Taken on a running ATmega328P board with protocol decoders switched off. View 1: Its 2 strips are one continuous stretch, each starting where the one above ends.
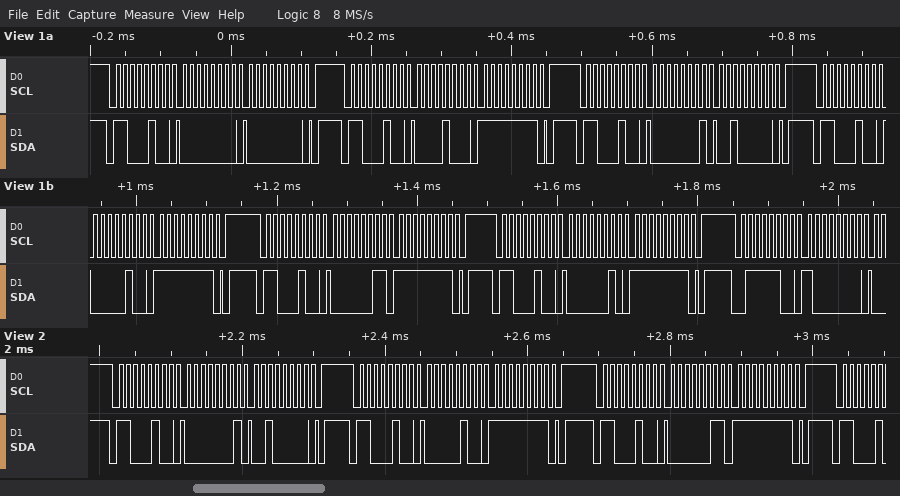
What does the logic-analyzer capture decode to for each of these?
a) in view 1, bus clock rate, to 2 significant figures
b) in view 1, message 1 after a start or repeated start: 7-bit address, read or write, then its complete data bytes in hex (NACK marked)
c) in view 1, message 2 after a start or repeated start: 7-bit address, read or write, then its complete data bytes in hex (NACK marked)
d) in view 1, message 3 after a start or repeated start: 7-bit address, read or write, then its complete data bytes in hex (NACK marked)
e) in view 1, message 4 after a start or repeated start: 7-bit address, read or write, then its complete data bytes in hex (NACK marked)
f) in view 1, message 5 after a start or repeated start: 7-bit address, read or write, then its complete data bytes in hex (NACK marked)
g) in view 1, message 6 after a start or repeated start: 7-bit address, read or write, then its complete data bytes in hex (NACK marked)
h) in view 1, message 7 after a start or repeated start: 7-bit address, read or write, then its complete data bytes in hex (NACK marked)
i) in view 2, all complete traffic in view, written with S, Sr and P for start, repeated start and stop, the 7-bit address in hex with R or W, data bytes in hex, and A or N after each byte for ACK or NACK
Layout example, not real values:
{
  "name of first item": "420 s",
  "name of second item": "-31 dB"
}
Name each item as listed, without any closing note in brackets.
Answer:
{
  "in view 1, bus clock rate, to 2 significant figures": "100 kHz",
  "in view 1, message 1 after a start or repeated start: 7-bit address, read or write, then its complete data bytes in hex": "0x62 write: 00 00",
  "in view 1, message 2 after a start or repeated start: 7-bit address, read or write, then its complete data bytes in hex": "0x62 write: 08 FF",
  "in view 1, message 3 after a start or repeated start: 7-bit address, read or write, then its complete data bytes in hex": "0x62 write: 01 20",
  "in view 1, message 4 after a start or repeated start: 7-bit address, read or write, then its complete data bytes in hex": "0x62 write: 04 FF",
  "in view 1, message 5 after a start or repeated start: 7-bit address, read or write, then its complete data bytes in hex": "0x62 write: 03 FF",
  "in view 1, message 6 after a start or repeated start: 7-bit address, read or write, then its complete data bytes in hex": "0x62 write: 02 FF",
  "in view 1, message 7 after a start or repeated start: 7-bit address, read or write, then its complete data bytes in hex": "0x3E write: 80",
  "in view 2, all complete traffic in view, written with S, Sr and P for start, repeated start and stop, the 7-bit address in hex with R or W, data bytes in hex, and A or N after each byte for ACK or NACK": "S 62W A 01 A 20 A P S 62W A 04 A FF A P S 62W A 03 A FF A P"
}
